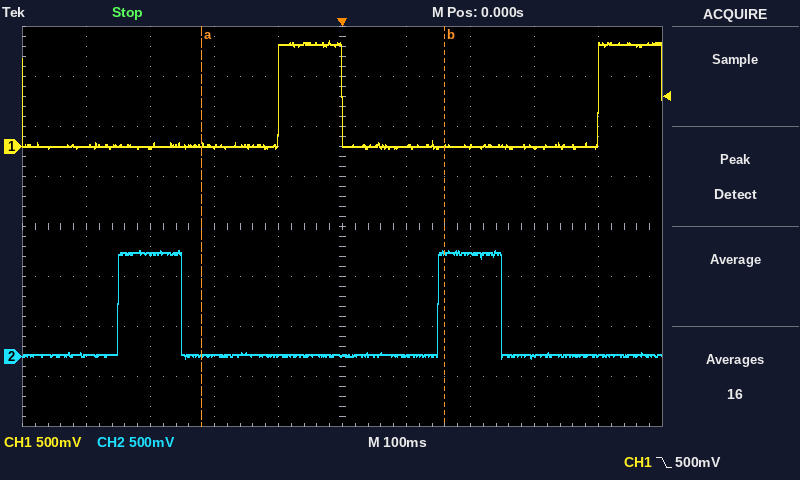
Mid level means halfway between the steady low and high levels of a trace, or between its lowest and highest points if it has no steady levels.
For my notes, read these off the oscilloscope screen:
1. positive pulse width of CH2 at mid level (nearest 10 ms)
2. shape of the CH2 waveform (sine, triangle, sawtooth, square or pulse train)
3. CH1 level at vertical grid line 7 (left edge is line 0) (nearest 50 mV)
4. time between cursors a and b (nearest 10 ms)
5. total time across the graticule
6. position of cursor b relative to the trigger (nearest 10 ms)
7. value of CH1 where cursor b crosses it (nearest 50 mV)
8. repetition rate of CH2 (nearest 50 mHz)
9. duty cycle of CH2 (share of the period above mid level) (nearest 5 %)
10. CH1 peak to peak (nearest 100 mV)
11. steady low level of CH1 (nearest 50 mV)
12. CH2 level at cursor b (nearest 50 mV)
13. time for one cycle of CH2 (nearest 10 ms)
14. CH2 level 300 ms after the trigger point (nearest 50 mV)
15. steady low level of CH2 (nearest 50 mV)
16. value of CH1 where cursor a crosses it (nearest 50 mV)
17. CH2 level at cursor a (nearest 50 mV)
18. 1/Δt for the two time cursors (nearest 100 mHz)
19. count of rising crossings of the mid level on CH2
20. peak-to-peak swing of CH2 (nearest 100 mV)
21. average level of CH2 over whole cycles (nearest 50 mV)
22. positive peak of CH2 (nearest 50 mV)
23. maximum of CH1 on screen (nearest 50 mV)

100 ms
pulse train
0 mV
380 ms
1 s
+160 ms
0 mV
2.00 Hz
20 %
1.10 V
0 mV
1.05 V
500 ms
0 mV
0 mV
0 mV
0 mV
2.6 Hz
2
1.10 V
200 mV
1.05 V
1.05 V
